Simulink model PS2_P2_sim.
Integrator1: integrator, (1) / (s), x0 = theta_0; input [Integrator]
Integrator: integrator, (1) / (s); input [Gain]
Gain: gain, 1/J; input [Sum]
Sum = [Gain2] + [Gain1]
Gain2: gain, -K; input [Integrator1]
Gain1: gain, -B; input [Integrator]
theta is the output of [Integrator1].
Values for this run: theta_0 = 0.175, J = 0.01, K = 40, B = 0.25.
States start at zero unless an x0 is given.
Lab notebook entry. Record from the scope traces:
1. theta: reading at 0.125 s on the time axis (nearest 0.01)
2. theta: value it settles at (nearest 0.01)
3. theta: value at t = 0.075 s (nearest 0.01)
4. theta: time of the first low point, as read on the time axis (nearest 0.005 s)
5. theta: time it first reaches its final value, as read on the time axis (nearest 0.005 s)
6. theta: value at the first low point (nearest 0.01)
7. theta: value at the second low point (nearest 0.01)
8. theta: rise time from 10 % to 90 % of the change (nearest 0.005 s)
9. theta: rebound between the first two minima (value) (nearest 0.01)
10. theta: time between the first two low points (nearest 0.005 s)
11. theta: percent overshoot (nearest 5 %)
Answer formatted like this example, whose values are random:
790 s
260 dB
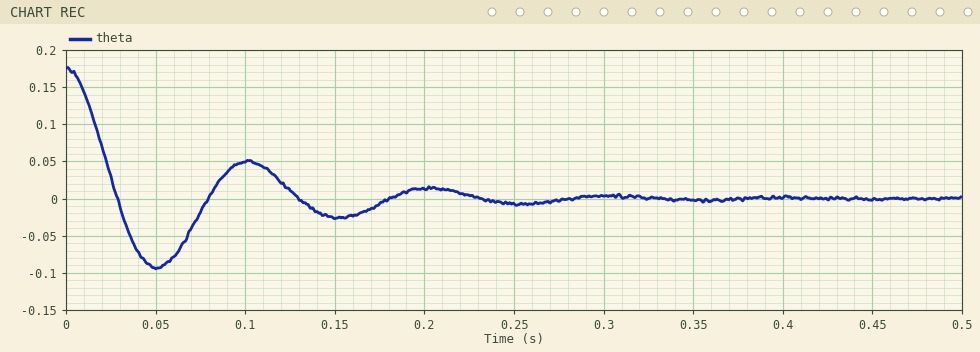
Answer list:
0.01
0.00
-0.02
0.050 s
0.030 s
-0.09
-0.03
0.020 s
0.05
0.100 s
55 %
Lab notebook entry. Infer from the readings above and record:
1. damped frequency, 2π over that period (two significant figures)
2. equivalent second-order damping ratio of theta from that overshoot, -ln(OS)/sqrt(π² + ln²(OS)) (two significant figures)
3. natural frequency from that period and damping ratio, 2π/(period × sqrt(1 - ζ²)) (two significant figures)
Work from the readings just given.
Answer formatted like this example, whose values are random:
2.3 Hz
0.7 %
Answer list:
63 rad/s
0.19
64 rad/s
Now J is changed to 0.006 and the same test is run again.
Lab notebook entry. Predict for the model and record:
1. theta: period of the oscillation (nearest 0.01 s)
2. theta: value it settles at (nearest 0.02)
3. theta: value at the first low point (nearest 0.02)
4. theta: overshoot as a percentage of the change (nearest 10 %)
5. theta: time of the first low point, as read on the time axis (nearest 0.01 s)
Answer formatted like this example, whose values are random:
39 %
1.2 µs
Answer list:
0.08 s
0.00
-0.08
40 %
0.04 s
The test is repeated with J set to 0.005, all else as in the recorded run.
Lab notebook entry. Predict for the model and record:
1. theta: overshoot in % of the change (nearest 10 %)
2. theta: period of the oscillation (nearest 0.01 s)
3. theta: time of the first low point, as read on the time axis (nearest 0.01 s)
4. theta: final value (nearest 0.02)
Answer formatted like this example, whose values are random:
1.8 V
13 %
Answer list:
40 %
0.07 s
0.04 s
0.00
